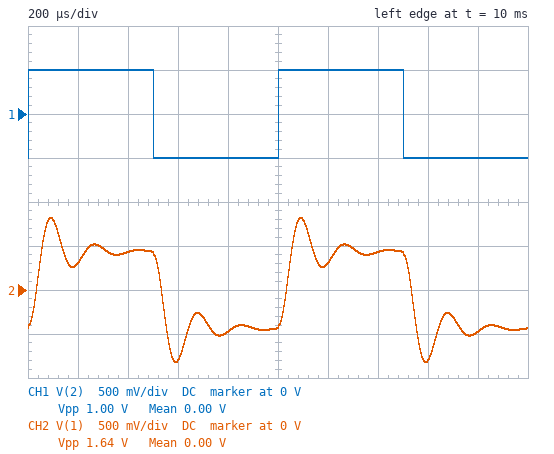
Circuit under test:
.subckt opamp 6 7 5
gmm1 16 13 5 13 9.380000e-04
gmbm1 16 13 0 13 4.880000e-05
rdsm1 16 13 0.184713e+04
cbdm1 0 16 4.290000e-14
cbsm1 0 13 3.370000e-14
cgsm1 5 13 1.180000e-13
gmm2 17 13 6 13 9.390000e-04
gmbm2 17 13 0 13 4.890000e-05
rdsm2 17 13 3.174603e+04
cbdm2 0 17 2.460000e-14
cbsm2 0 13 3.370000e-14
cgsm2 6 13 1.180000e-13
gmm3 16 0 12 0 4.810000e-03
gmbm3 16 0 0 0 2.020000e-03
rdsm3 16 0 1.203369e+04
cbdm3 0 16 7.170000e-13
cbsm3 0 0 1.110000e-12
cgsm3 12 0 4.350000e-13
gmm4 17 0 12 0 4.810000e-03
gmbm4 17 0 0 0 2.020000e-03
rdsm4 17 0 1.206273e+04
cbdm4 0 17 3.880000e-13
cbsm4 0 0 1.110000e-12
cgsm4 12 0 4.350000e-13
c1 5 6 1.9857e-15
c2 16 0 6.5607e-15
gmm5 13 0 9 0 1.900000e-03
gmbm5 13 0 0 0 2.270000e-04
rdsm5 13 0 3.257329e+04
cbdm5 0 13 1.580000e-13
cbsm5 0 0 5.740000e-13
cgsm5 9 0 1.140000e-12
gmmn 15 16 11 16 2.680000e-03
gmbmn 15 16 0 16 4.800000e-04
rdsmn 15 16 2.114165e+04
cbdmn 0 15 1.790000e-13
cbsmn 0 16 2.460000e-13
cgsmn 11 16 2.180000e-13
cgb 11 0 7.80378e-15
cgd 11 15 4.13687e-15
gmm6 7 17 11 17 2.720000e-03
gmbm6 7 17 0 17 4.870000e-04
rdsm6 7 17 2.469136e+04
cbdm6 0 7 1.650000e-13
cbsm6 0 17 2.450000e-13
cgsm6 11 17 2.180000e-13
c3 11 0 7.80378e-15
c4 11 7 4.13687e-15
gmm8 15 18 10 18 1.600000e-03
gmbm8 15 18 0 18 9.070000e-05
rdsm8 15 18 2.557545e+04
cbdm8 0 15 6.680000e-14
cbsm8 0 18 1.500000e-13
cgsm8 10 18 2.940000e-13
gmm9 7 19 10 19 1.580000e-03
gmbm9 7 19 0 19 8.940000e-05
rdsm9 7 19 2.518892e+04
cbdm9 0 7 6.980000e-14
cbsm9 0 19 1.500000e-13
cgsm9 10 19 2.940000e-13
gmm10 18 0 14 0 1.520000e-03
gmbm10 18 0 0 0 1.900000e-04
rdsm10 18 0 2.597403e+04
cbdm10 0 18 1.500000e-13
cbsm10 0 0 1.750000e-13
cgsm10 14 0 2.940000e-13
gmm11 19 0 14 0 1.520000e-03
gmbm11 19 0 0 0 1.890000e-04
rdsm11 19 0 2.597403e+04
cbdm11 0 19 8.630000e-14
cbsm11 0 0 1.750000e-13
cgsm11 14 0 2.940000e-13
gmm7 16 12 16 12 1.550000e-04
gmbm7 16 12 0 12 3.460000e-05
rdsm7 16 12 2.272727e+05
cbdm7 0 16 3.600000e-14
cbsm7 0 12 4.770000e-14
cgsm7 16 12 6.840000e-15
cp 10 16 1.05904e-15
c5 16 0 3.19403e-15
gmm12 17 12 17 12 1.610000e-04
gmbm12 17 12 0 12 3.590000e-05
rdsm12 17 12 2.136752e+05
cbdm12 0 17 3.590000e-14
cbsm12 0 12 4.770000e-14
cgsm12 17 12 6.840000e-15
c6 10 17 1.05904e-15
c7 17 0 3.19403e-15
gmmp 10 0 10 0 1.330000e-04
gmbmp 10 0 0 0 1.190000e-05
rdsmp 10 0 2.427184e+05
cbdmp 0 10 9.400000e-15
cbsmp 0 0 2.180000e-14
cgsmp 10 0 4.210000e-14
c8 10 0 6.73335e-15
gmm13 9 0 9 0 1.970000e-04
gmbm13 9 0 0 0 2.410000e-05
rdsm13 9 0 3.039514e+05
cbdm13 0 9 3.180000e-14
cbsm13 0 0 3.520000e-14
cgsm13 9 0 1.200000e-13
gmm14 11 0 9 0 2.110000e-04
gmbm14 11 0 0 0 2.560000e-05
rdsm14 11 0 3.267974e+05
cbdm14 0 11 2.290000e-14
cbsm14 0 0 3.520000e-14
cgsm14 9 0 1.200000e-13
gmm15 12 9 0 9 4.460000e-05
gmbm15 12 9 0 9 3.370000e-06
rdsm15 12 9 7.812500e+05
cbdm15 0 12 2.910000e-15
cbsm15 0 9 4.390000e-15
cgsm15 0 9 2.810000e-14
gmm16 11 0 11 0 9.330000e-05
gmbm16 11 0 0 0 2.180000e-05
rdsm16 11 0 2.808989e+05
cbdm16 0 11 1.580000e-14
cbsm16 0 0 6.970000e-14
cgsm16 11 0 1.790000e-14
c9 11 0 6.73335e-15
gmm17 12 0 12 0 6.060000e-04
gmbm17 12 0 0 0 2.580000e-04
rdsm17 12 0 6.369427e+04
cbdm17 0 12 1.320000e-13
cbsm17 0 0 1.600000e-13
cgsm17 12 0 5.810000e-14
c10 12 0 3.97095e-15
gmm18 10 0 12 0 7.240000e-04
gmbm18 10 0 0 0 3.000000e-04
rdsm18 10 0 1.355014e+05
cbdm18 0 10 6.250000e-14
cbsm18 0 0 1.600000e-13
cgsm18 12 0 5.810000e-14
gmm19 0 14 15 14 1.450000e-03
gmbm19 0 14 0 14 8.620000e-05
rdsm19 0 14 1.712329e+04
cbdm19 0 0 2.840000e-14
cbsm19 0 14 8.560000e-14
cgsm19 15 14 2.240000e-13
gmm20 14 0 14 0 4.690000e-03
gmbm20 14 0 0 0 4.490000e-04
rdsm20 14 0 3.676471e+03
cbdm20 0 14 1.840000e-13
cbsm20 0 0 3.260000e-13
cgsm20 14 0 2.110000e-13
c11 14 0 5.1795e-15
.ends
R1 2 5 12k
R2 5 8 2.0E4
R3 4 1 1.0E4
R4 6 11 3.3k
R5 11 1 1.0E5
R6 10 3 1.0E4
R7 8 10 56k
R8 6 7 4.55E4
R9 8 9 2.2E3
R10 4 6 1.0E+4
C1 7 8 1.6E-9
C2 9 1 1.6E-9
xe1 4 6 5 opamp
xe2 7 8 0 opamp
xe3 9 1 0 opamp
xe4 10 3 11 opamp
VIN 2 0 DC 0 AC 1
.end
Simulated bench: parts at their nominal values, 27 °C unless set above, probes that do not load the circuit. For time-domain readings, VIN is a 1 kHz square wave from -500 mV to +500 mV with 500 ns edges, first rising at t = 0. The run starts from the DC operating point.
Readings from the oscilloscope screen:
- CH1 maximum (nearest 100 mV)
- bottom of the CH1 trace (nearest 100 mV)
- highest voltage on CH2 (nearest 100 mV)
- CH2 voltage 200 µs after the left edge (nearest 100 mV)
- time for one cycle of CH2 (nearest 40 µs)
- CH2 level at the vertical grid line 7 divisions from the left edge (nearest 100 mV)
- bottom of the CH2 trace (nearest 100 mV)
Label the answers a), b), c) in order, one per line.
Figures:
a) 500 mV
b) -500 mV
c) 800 mV
d) 300 mV
e) 1.00 ms
f) 400 mV
g) -800 mV
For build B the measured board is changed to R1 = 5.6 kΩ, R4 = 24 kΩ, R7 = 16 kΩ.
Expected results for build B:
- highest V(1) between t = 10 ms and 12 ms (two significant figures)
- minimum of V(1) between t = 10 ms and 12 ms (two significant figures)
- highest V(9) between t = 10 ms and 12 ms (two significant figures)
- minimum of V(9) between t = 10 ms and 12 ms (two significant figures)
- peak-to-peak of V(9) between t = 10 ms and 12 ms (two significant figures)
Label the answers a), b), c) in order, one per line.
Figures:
a) 1.1 V
b) -1.1 V
c) 100 mV
d) -100 mV
e) 210 mV
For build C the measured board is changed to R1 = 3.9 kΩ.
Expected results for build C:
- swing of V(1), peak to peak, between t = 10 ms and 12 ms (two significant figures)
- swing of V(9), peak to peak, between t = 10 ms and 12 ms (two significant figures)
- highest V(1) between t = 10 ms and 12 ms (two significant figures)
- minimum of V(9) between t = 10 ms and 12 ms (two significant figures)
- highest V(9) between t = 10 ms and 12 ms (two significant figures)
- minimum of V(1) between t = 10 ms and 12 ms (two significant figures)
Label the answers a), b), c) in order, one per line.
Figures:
a) 2.3 V
b) 230 mV
c) 1.2 V
d) -110 mV
e) 110 mV
f) -1.2 V
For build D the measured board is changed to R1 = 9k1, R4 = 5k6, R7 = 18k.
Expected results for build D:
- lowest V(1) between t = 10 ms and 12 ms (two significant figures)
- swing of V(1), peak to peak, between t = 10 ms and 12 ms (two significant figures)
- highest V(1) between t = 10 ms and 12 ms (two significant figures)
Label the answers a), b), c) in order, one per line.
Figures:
a) -940 mV
b) 1.9 V
c) 940 mV
